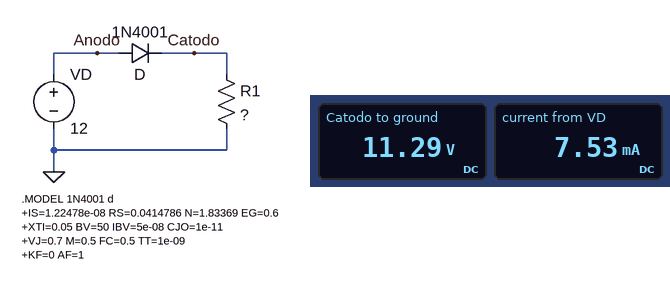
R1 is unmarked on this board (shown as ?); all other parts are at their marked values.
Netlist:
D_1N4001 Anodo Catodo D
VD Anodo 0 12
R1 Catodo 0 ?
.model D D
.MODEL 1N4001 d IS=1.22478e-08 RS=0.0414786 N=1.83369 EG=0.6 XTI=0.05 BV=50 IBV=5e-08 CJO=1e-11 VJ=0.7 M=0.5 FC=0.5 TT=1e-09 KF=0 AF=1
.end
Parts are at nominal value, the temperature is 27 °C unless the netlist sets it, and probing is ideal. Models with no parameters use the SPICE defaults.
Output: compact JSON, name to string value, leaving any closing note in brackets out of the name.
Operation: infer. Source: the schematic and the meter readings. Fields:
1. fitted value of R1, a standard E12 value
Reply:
{"fitted value of R1, a standard E12 value": "1.5 kΩ"}
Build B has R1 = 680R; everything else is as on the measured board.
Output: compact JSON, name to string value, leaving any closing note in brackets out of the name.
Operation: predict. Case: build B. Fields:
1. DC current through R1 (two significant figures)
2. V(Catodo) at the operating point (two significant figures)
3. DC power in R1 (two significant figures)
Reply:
{"DC current through R1": "17 mA", "V(Catodo) at the operating point": "11 V", "DC power in R1": "190 mW"}
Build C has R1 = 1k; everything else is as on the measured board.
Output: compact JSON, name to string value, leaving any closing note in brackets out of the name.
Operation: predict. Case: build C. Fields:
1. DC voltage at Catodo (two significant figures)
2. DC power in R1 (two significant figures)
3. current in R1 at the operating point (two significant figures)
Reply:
{"DC voltage at Catodo": "11 V", "DC power in R1": "130 mW", "current in R1 at the operating point": "11 mA"}
